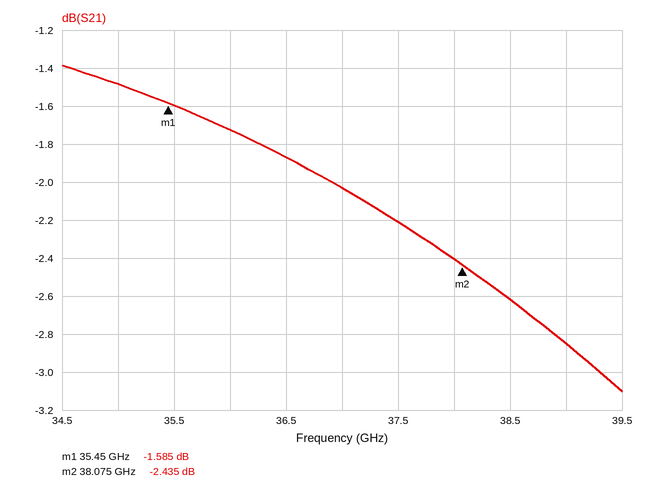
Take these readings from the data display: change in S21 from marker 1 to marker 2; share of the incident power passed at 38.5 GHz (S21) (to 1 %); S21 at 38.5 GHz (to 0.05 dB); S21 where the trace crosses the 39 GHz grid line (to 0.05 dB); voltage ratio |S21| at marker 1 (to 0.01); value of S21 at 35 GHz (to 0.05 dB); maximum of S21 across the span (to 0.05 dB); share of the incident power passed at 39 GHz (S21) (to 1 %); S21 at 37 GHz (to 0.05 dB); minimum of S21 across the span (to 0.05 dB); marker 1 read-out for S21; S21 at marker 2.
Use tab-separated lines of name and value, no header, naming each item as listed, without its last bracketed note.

change in S21 from marker 1 to marker 2	-0.850 dB
share of the incident power passed at 38.5 GHz (S21)	55 %
S21 at 38.5 GHz	-2.60 dB
S21 where the trace crosses the 39 GHz grid line	-2.85 dB
voltage ratio |S21| at marker 1	0.83
value of S21 at 35 GHz	-1.50 dB
maximum of S21 across the span	-1.40 dB
share of the incident power passed at 39 GHz (S21)	52 %
S21 at 37 GHz	-2.05 dB
minimum of S21 across the span	-3.10 dB
marker 1 read-out for S21	-1.585 dB
S21 at marker 2	-2.435 dB
